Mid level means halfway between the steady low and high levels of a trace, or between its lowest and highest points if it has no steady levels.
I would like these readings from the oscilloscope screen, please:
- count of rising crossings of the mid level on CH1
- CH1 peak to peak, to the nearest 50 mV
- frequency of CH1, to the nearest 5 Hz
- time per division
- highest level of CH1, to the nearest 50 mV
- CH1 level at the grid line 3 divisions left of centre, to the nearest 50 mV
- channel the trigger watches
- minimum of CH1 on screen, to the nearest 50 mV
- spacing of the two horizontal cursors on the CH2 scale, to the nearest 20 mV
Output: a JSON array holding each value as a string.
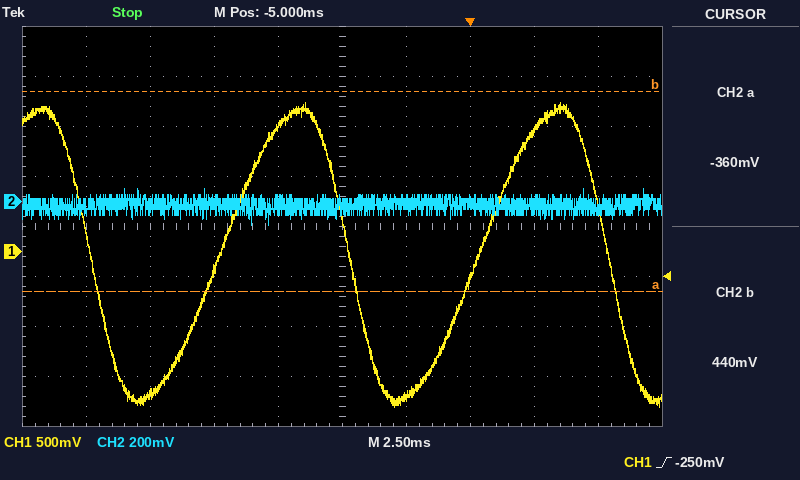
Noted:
["2", "3.05 V", "100 Hz", "2.5 ms", "1.50 V", "-1.40 V", "CH1", "-1.55 V", "800 mV"]
